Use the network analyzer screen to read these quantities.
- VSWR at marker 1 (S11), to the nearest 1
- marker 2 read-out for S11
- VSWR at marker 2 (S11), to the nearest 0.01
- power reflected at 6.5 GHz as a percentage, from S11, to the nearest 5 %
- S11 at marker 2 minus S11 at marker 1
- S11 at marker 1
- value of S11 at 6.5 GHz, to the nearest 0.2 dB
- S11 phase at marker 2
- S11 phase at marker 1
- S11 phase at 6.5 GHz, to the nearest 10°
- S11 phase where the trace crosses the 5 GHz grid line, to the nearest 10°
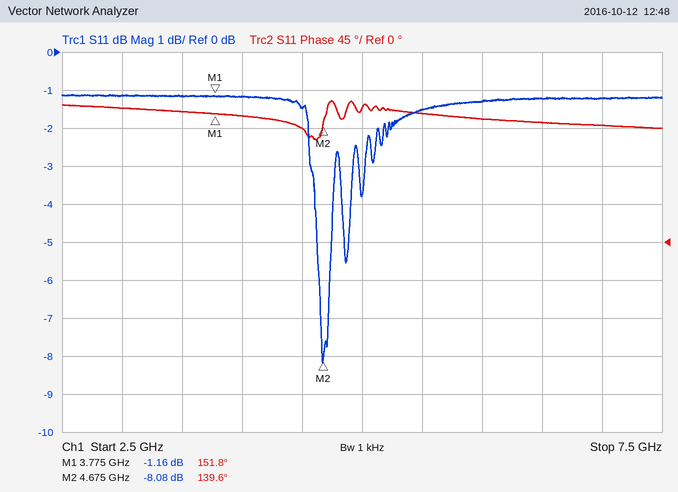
15
-8.08 dB
2.30
75 %
-6.92 dB
-1.16 dB
-1.2 dB
139.6°
151.8°
140°
160°
